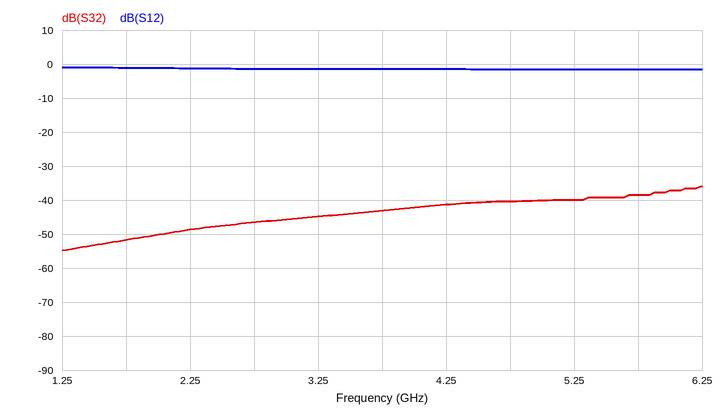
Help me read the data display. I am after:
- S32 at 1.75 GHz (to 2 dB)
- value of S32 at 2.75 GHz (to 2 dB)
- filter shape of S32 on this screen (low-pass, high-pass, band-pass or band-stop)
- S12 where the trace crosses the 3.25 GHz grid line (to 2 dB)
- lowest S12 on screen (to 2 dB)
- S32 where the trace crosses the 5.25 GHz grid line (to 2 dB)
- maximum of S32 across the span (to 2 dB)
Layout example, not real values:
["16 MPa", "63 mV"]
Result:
["-52 dB", "-46 dB", "high-pass", "-2 dB", "-2 dB", "-40 dB", "-36 dB"]
